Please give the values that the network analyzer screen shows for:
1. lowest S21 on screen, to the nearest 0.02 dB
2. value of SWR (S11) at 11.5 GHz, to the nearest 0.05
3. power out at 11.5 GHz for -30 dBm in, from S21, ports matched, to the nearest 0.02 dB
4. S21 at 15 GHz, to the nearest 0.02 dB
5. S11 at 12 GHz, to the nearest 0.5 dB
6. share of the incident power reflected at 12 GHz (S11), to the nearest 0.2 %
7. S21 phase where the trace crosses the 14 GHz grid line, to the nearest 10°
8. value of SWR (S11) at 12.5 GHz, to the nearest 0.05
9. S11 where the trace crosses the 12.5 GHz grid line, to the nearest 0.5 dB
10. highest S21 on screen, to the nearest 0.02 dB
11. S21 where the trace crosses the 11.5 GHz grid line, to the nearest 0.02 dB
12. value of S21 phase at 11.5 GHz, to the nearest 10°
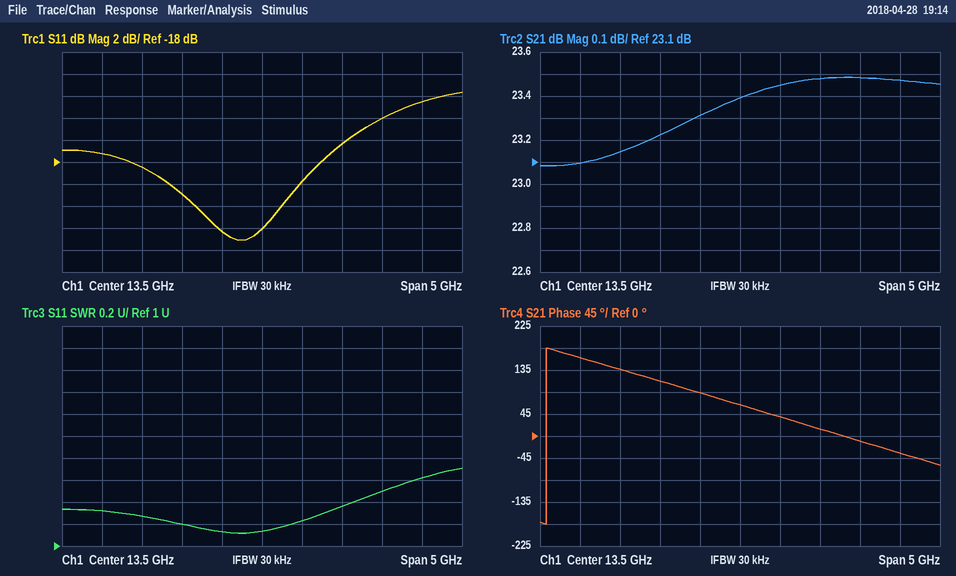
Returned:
23.08 dB
1.30
-6.90 dBm
23.48 dB
-18.5 dB
1.4 %
40°
1.20
-21.0 dB
23.48 dB
23.10 dB
160°
